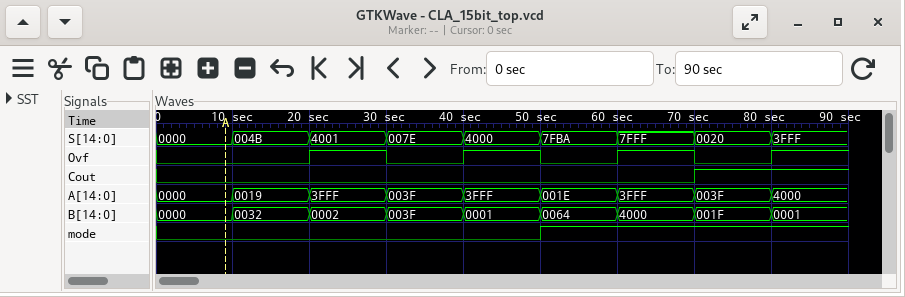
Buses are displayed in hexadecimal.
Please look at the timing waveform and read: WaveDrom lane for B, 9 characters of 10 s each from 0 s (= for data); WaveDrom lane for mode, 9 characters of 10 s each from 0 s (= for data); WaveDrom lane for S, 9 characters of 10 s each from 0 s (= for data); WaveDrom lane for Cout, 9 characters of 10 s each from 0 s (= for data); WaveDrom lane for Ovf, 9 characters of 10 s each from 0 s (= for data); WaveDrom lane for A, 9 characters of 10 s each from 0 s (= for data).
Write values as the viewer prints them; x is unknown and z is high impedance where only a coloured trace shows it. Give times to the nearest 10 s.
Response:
{name: 'B', wave: '=========', data: '0000 0032 0002 003F 0001 0064 4000 001F 0001'}
{name: 'mode', wave: '0....1...'}
{name: 'S', wave: '=========', data: '0000 004B 4001 007E 4000 7FBA 7FFF 0020 3FFF'}
{name: 'Cout', wave: '0......1.'}
{name: 'Ovf', wave: '0.1010101'}
{name: 'A', wave: '=========', data: '0000 0019 3FFF 003F 3FFF 001E 3FFF 003F 4000'}
